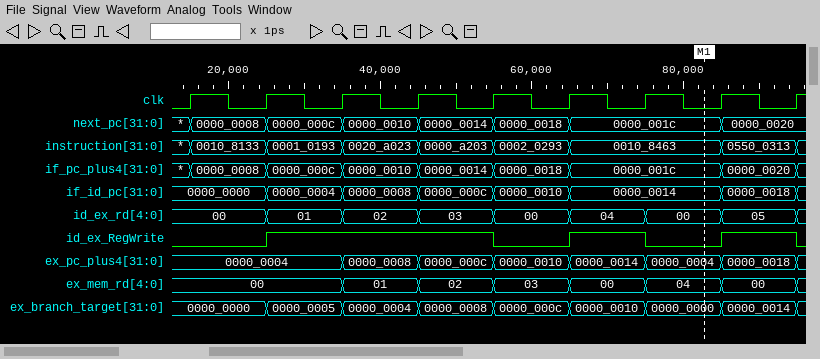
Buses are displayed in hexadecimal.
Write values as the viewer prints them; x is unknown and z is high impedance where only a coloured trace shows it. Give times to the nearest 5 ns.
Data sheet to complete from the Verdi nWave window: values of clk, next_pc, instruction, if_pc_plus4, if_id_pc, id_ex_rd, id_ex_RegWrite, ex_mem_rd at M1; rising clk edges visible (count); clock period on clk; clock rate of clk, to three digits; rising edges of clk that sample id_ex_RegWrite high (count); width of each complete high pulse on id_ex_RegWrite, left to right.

clk=0, next_pc=0000_001c, instruction=0010_8463, if_pc_plus4=0000_001c, if_id_pc=0000_0014, id_ex_rd=00, id_ex_RegWrite=0, ex_mem_rd=04
9
10 ns
100 MHz
5
30 ns, 10 ns, 10 ns
